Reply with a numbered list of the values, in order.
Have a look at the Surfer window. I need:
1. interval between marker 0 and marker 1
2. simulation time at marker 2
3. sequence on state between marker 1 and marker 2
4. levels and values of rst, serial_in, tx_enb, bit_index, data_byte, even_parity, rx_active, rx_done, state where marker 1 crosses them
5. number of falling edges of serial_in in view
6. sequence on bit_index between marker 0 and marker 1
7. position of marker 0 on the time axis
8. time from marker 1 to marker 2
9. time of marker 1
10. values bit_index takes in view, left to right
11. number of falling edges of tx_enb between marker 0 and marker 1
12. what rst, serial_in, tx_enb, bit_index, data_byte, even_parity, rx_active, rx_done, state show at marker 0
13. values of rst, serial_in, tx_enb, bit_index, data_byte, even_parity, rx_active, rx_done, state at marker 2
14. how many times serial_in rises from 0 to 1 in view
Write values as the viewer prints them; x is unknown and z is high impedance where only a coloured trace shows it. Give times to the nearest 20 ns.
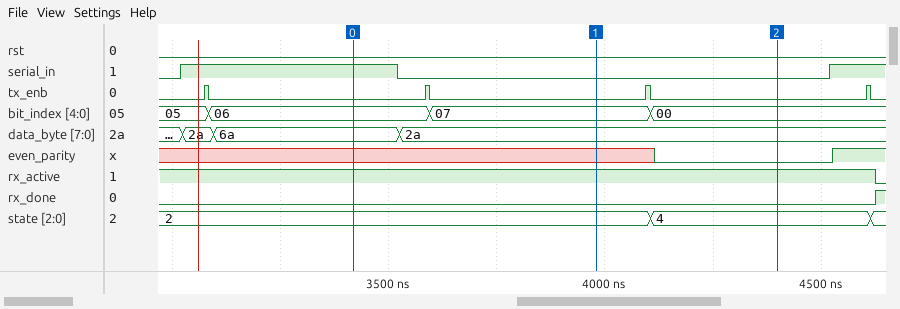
1. 560 ns
2. 4400 ns
3. 2, 4
4. rst=0, serial_in=0, tx_enb=0, bit_index=07, data_byte=2a, even_parity=x, rx_active=1, rx_done=0, state=2
5. 1
6. 06, 07
7. 3420 ns
8. 420 ns
9. 3980 ns
10. 05, 06, 07, 00
11. 1
12. rst=0, serial_in=1, tx_enb=0, bit_index=06, data_byte=6a, even_parity=x, rx_active=1, rx_done=0, state=2
13. rst=0, serial_in=0, tx_enb=0, bit_index=00, data_byte=2a, even_parity=0, rx_active=1, rx_done=0, state=4
14. 2
